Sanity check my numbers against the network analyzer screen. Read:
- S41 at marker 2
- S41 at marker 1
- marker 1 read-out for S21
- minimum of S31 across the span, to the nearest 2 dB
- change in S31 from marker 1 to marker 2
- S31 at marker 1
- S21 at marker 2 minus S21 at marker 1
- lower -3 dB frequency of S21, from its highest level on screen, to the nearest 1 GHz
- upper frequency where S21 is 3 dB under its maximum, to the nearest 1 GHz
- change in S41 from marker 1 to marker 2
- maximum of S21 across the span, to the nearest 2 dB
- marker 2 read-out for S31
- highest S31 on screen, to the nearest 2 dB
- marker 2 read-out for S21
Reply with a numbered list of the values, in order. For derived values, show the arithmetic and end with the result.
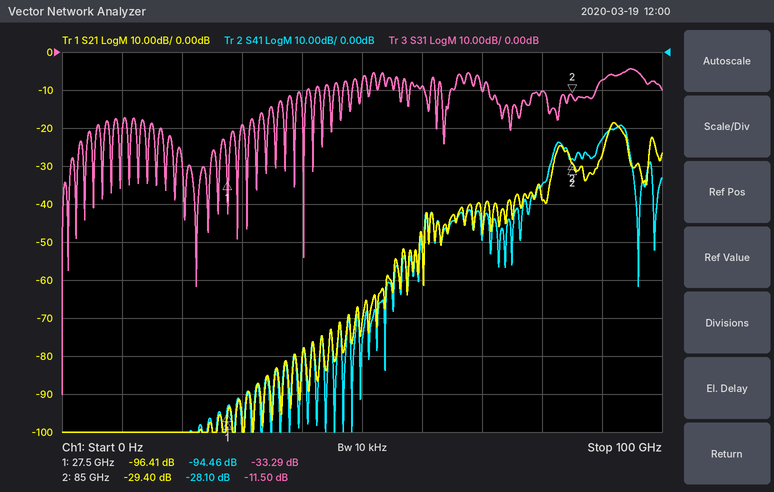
1. -28.10 dB
2. -94.46 dB
3. -96.41 dB
4. -90 dB
5. -11.5 − (-33.29) = 21.79 dB
6. -33.29 dB
7. -29.4 − (-96.41) = 67.01 dB
8. 91 GHz
9. 94 GHz
10. -28.1 − (-94.46) = 66.36 dB
11. -18 dB
12. -11.50 dB
13. -4 dB
14. -29.40 dB
